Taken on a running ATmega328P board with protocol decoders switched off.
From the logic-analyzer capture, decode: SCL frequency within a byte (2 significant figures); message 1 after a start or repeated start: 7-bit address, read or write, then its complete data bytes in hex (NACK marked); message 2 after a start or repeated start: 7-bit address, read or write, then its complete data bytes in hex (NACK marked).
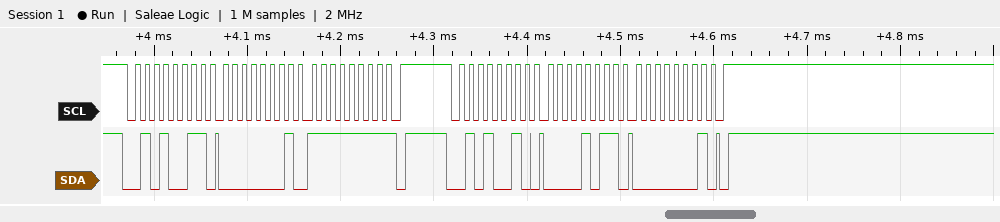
100 kHz
0x29 read: 01 FF NACK
0x29 write: 0B 01
